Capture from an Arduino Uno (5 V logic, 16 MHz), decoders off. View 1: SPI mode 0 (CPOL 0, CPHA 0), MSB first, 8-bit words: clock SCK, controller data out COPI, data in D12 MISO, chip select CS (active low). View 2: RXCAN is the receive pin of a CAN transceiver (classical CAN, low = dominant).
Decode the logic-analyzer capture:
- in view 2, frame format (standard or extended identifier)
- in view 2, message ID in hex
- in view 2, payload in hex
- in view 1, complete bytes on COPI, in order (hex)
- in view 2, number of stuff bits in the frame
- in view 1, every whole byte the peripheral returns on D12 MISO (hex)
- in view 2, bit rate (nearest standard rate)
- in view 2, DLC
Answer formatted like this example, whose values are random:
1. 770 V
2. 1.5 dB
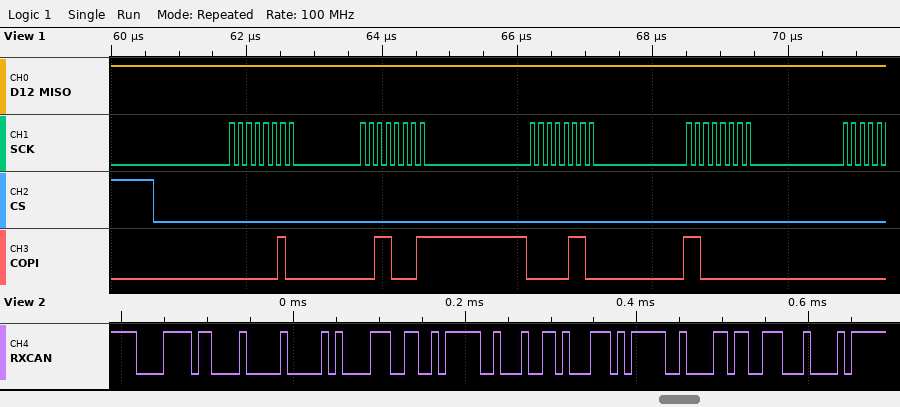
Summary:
1. standard
2. 0x0F6
3. 00 87 32 FA 26 8E BE 86
4. 02 31 06 C0
5. 4
6. FF FF FF FF
7. 125 kbit/s
8. 8
